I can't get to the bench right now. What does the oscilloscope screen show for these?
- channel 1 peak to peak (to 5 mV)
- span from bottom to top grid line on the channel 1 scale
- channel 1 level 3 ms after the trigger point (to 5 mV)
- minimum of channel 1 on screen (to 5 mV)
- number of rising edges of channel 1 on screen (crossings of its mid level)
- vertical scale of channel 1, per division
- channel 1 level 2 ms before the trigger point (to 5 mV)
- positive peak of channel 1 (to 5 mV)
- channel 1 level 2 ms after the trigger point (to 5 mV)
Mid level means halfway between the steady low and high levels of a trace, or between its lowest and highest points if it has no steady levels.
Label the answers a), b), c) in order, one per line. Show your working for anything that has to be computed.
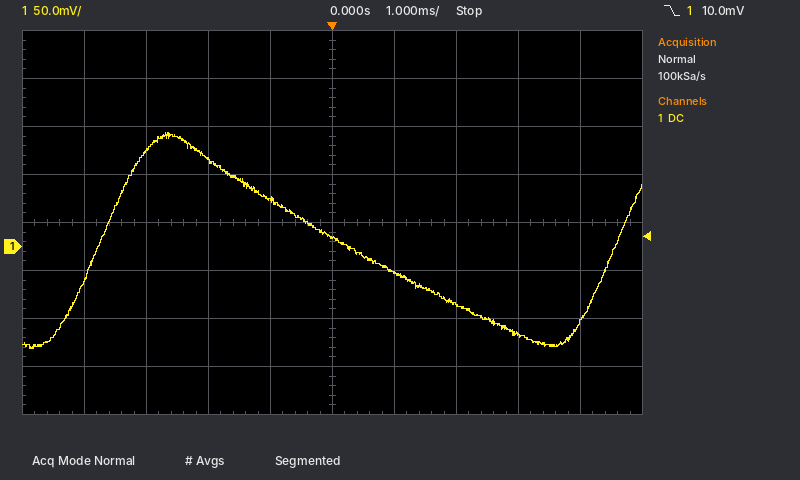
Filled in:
a) 120 mV − (-105 mV) = 225 mV
b) 400 mV
c) -90 mV
d) -105 mV
e) 2
f) 50 mV
g) 90 mV
h) 120 mV
i) -60 mV
